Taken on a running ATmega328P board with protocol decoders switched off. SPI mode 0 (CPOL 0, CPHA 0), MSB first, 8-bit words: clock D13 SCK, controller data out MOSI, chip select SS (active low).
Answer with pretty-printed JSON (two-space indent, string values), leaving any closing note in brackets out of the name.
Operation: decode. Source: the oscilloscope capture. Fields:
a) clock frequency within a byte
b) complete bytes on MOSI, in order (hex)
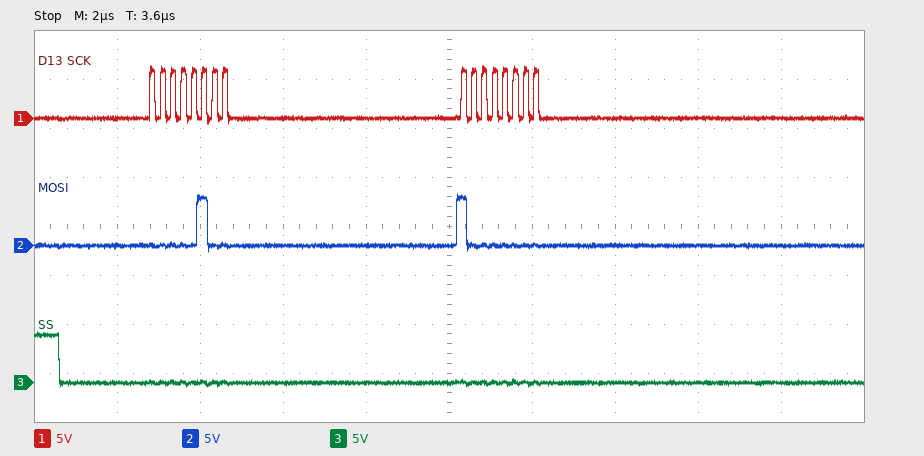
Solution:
{
  "clock frequency within a byte": "4 MHz",
  "complete bytes on MOSI, in order": "0x04 0x80"
}
